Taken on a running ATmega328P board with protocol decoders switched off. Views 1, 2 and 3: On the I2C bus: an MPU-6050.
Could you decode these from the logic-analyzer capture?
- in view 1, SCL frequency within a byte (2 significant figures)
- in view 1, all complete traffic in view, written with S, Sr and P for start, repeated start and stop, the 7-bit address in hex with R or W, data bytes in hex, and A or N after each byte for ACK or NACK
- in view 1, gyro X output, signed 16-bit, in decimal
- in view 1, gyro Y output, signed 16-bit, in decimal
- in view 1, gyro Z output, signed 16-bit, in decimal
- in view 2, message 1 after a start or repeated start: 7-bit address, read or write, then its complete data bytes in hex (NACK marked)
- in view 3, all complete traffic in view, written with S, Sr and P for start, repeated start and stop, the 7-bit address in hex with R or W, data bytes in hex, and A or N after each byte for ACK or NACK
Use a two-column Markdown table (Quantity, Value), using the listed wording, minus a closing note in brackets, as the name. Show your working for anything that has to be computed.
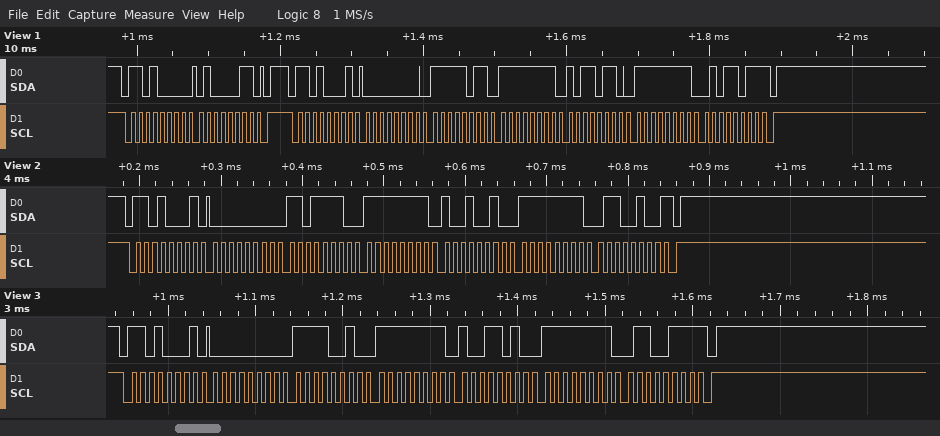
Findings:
| Quantity | Value |
|---|---|
| in view 1, SCL frequency within a byte | 100 kHz |
| in view 1, all complete traffic in view, written with S, Sr and P for start, repeated start and stop, the 7-bit address in hex with R or W, data bytes in hex, and A or N after each byte for ACK or NACK | S 68W A 43 A P S 68R A 00 A FB A FF A B6 A FF A 5B N P |
| in view 1, gyro X output, signed 16-bit, in decimal | 0x00FB = 251 |
| in view 1, gyro Y output, signed 16-bit, in decimal | 0xFFB6 = -74 |
| in view 1, gyro Z output, signed 16-bit, in decimal | 0xFF5B = -165 |
| in view 2, message 1 after a start or repeated start: 7-bit address, read or write, then its complete data bytes in hex | 0x68 read: 00 DE FF 92 FF 64 NACK |
| in view 3, all complete traffic in view, written with S, Sr and P for start, repeated start and stop, the 7-bit address in hex with R or W, data bytes in hex, and A or N after each byte for ACK or NACK | S 68R A 00 A F2 A FF A 9A A FF A 67 N P |
